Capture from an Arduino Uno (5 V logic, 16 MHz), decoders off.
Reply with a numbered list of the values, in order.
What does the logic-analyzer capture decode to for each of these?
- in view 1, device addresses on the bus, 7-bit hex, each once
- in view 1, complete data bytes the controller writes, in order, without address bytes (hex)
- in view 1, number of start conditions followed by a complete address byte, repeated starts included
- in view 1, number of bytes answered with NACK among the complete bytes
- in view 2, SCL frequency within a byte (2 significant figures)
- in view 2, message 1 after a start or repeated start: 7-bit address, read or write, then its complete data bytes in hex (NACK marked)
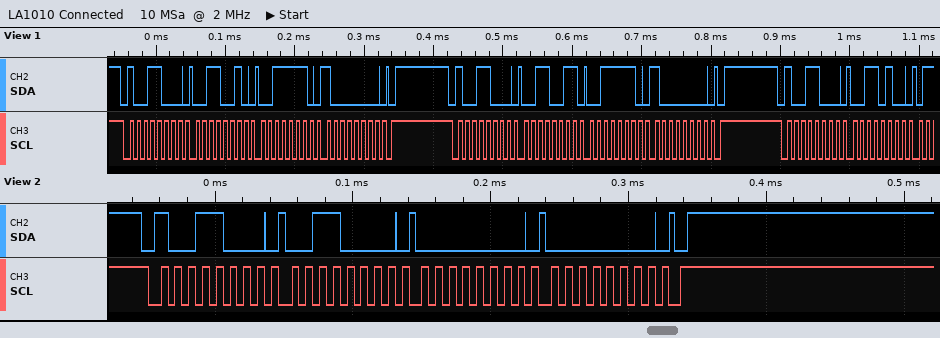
1. 0x4C
2. 32 3E 80 33 3E 80 34
3. 3
4. 0
5. 100 kHz
6. 0x4C write: 30 00 00
